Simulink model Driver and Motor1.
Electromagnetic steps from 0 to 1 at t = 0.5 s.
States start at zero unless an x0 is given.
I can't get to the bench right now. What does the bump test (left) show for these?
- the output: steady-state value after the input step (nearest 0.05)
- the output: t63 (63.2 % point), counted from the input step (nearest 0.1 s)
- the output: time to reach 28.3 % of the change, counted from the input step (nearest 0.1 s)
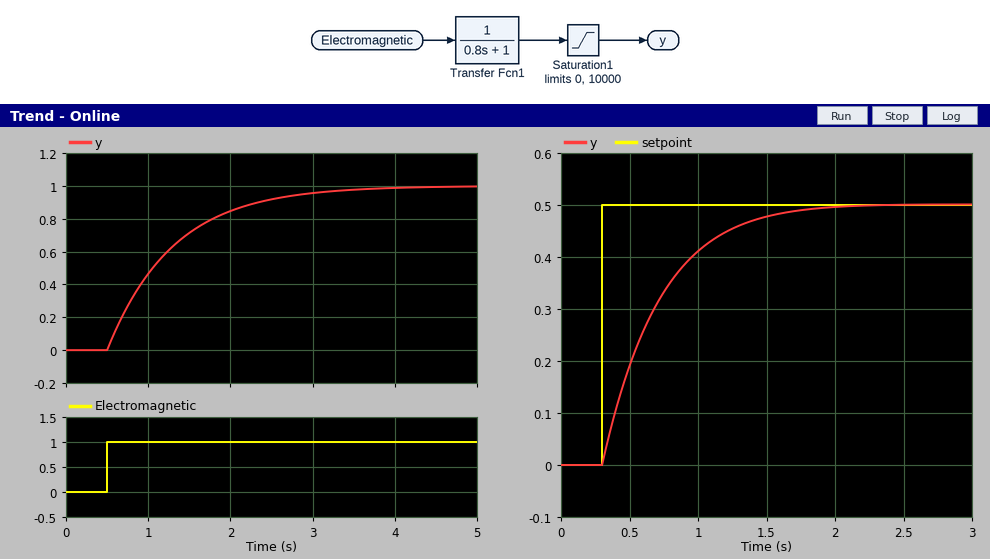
1.00
0.8 s
0.3 s
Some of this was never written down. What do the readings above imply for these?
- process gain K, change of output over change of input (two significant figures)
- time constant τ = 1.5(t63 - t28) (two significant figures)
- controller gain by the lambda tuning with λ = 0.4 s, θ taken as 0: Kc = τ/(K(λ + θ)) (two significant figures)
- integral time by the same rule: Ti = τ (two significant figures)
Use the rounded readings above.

1.0
0.75 s
1.9
0.75 s
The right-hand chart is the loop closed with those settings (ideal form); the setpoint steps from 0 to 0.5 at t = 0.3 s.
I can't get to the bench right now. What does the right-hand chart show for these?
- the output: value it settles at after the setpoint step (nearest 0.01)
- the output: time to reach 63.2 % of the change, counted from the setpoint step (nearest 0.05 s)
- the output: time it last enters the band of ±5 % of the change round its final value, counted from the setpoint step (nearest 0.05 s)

0.50
0.40 s
1.15 s
